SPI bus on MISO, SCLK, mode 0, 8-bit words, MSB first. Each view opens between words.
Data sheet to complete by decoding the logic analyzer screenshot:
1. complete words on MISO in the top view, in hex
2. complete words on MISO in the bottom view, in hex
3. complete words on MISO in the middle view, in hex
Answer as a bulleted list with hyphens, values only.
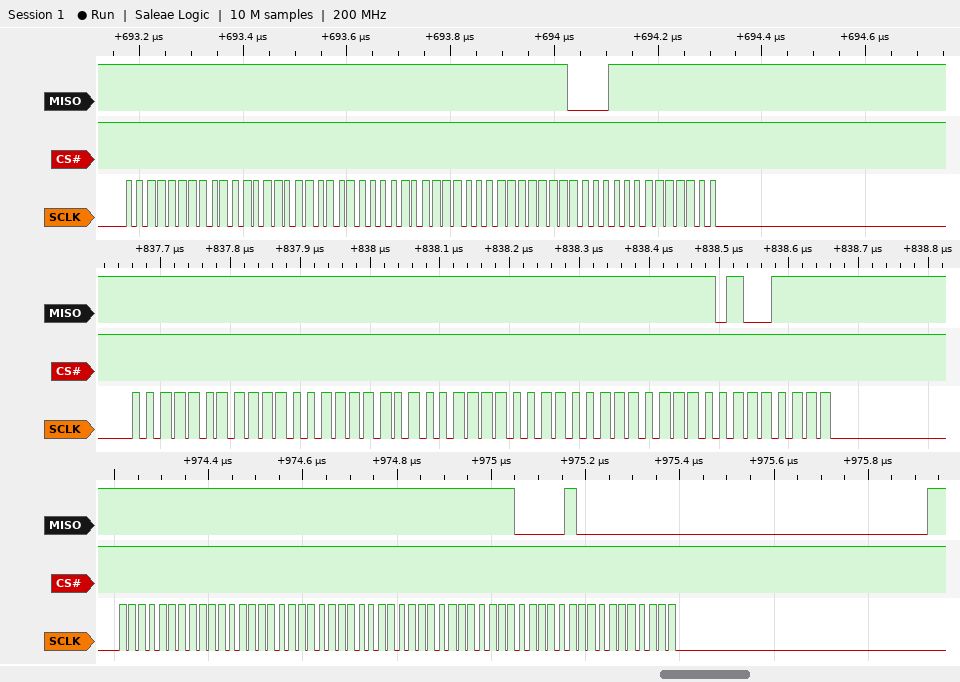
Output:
- FF, FF, FF, FF, FF, C3, FF
- FF, FF, FF, FF, FF, 04, 00
- FF, FF, FF, FF, FF, 4F
